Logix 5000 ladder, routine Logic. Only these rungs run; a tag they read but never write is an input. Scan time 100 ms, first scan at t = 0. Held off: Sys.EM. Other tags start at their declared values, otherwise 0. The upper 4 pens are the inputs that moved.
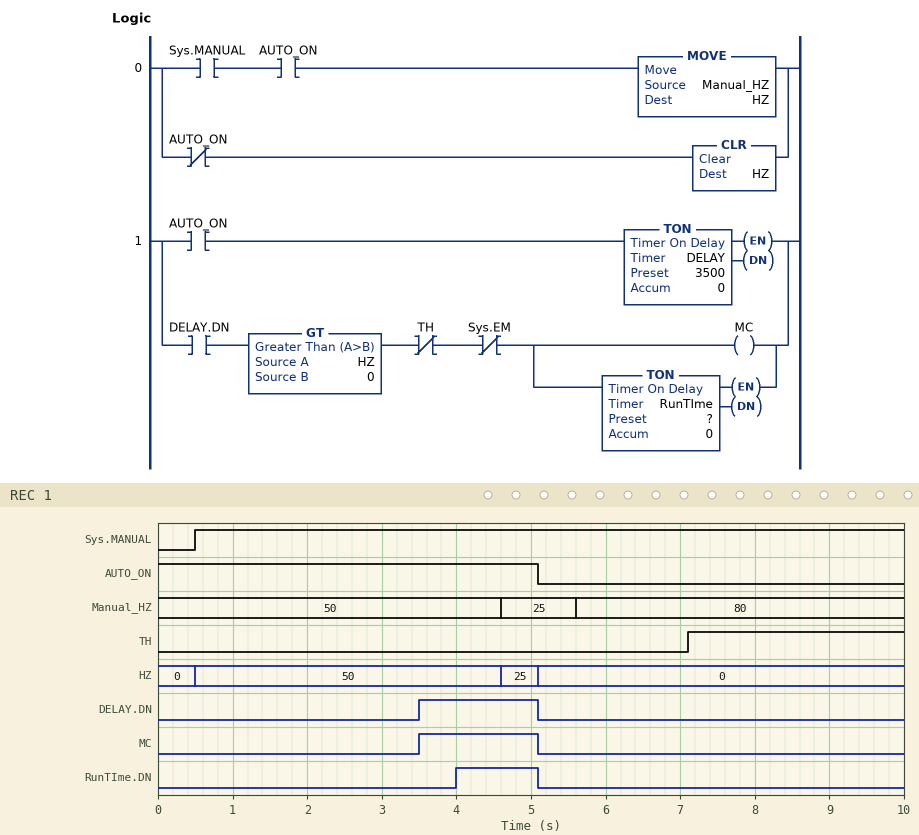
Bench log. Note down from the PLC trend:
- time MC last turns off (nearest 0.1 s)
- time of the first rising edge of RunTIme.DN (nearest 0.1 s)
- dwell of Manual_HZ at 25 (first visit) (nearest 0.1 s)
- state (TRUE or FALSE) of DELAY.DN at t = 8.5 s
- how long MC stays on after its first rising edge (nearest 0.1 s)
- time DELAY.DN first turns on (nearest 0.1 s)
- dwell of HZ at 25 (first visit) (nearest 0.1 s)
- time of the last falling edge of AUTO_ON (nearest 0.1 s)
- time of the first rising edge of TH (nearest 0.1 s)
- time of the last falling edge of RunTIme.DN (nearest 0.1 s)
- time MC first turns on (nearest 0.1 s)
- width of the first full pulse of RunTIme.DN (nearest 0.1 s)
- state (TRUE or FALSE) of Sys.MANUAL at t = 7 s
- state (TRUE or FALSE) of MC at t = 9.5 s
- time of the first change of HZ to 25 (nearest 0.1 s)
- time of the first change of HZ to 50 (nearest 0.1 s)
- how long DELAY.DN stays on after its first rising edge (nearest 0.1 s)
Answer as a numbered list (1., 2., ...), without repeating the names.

1. 5.1 s
2. 4.0 s
3. 1.0 s
4. FALSE
5. 1.6 s
6. 3.5 s
7. 0.5 s
8. 5.1 s
9. 7.1 s
10. 5.1 s
11. 3.5 s
12. 1.1 s
13. TRUE
14. FALSE
15. 4.6 s
16. 0.5 s
17. 1.6 s
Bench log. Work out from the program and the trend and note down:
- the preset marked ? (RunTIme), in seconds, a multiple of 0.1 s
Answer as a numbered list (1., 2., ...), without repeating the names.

1. 0.5 s
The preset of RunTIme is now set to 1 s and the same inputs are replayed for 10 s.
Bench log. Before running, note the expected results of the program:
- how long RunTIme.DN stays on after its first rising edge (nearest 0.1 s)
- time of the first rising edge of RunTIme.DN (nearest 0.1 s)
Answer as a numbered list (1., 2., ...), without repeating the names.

1. 0.6 s
2. 4.5 s
